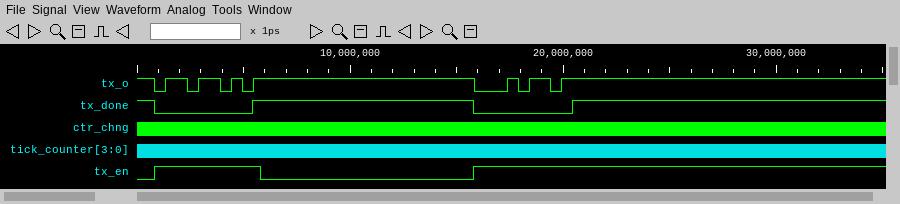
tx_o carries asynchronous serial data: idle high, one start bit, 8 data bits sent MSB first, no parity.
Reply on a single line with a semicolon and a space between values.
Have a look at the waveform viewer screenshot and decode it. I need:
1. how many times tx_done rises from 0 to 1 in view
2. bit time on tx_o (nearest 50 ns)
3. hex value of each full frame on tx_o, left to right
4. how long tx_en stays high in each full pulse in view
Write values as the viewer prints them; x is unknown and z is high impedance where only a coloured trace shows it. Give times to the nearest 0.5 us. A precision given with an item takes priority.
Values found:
2; 500 ns; DA, 2D; 5 us
